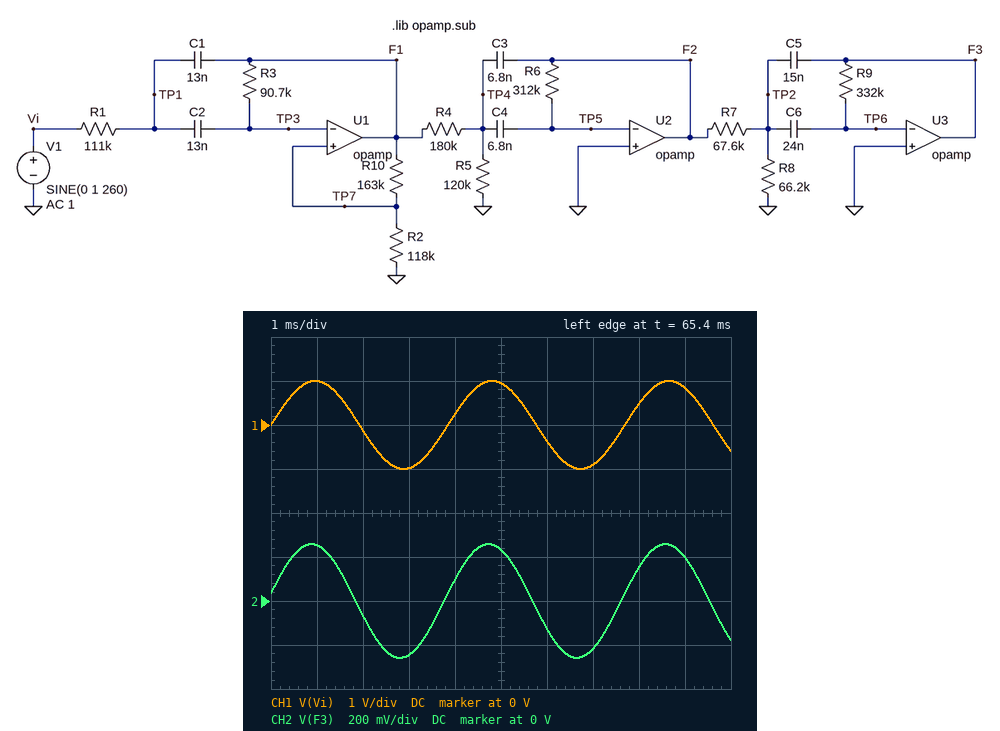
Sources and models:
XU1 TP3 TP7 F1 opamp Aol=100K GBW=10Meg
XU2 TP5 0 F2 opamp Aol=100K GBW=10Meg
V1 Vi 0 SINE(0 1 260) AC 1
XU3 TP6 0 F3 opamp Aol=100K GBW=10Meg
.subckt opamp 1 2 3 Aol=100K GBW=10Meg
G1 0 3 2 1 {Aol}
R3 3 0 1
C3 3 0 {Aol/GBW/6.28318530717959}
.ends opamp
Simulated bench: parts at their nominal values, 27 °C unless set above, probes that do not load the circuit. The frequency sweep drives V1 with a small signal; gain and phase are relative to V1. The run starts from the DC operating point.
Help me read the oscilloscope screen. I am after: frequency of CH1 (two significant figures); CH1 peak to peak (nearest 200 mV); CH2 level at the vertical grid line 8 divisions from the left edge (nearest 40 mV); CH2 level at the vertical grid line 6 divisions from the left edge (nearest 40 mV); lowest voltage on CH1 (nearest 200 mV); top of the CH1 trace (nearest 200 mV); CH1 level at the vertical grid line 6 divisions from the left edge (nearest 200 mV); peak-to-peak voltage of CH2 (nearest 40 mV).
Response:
260 Hz
2.0 V
160 mV
-120 mV
-1.0 V
1.0 V
-400 mV
520 mV
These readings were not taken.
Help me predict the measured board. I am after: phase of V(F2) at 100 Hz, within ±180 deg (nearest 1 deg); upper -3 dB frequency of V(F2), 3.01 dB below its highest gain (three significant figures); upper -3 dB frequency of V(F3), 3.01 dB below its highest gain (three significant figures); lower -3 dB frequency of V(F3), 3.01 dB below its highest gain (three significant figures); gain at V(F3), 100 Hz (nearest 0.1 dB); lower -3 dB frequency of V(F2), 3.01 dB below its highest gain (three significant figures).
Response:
58 deg
210 Hz
153 Hz
73.5 Hz
3.5 dB
98.4 Hz
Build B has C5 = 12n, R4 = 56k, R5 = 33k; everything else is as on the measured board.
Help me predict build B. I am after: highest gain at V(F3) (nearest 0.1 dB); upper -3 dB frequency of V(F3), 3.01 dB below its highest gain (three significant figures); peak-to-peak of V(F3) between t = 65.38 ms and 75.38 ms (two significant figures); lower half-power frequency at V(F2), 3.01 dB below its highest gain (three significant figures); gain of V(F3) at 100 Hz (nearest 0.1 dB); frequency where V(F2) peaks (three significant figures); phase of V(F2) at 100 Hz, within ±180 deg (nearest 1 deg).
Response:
4.6 dB
297 Hz
2.9 V
195 Hz
4.3 dB
274 Hz
93 deg
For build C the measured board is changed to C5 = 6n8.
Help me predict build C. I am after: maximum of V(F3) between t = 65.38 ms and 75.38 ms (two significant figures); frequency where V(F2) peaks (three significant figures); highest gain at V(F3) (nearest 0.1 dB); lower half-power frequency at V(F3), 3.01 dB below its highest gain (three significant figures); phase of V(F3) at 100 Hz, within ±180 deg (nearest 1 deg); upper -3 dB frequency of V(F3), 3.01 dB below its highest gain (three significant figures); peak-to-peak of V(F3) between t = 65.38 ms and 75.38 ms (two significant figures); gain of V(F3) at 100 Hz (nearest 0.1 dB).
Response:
610 mV
146 Hz
9.5 dB
99.9 Hz
-98 deg
171 Hz
1.2 V
6.5 dB
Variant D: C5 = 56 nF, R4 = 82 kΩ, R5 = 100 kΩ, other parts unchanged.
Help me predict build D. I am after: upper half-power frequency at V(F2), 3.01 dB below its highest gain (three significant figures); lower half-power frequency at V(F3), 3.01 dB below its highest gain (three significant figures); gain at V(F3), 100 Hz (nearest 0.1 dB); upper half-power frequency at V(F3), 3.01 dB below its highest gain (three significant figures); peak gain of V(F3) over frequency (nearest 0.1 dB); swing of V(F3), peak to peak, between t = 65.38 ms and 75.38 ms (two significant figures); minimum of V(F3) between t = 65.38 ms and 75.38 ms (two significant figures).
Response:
247 Hz
53.6 Hz
-7.8 dB
210 Hz
-7.1 dB
350 mV
-170 mV
